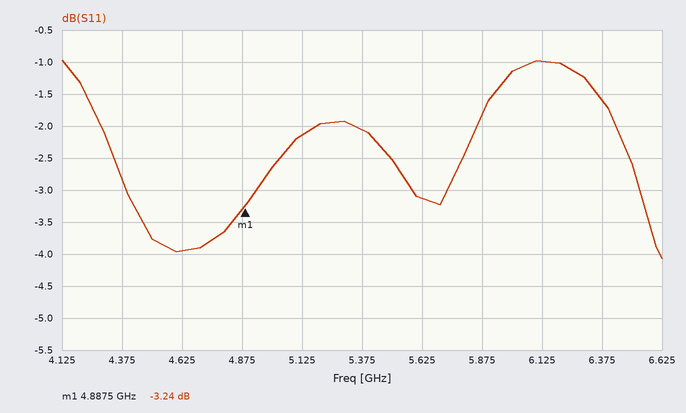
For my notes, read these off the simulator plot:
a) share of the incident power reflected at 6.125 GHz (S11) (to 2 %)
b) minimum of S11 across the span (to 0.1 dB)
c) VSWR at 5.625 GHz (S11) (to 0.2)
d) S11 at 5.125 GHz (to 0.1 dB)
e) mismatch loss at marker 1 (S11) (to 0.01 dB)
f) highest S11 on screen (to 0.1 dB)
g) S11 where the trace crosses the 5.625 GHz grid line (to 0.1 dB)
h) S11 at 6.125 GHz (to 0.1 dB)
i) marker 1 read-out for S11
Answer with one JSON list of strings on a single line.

["80 %", "-4.1 dB", "5.6", "-2.1 dB", "2.79 dB", "-1.0 dB", "-3.1 dB", "-1.0 dB", "-3.24 dB"]
